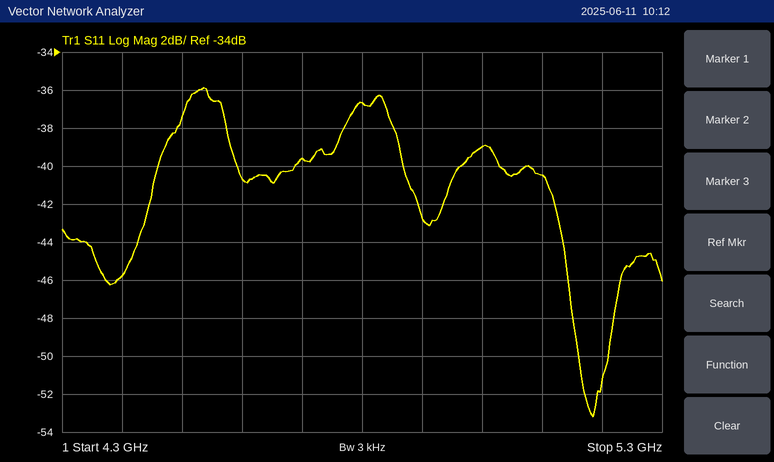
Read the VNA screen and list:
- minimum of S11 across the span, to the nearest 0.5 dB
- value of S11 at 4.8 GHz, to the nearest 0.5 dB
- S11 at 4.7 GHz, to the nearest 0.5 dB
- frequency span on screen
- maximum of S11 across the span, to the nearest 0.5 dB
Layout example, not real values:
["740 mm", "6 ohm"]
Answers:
["-53.0 dB", "-36.5 dB", "-39.5 dB", "1 GHz", "-36.0 dB"]
